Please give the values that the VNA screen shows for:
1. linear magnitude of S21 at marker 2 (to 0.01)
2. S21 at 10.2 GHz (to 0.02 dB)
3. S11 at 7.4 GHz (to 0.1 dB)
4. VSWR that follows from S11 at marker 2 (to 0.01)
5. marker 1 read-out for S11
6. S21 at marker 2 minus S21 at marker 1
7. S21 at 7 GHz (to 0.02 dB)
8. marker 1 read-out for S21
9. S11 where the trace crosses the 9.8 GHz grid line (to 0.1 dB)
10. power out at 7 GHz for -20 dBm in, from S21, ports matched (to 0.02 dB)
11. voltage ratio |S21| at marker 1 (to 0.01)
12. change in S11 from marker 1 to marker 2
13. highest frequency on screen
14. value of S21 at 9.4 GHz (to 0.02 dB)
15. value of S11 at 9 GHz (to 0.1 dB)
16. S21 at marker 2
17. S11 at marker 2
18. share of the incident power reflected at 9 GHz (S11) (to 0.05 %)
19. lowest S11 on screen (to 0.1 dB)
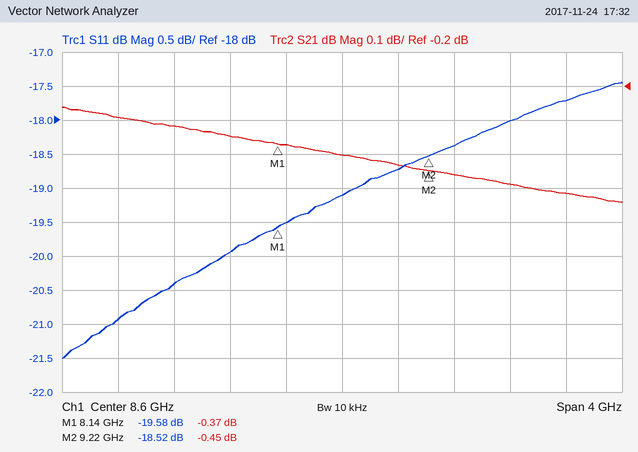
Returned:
0.95
-0.52 dB
-20.4 dB
1.27
-19.58 dB
-0.08 dB
-0.30 dB
-0.37 dB
-18.0 dB
-20.30 dBm
0.96
1.06 dB
10.6 GHz
-0.46 dB
-18.7 dB
-0.45 dB
-18.52 dB
1.35 %
-21.5 dB
